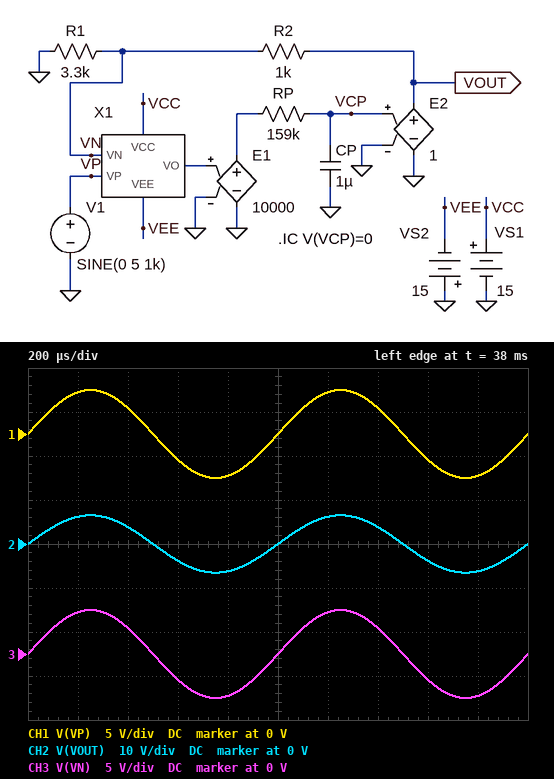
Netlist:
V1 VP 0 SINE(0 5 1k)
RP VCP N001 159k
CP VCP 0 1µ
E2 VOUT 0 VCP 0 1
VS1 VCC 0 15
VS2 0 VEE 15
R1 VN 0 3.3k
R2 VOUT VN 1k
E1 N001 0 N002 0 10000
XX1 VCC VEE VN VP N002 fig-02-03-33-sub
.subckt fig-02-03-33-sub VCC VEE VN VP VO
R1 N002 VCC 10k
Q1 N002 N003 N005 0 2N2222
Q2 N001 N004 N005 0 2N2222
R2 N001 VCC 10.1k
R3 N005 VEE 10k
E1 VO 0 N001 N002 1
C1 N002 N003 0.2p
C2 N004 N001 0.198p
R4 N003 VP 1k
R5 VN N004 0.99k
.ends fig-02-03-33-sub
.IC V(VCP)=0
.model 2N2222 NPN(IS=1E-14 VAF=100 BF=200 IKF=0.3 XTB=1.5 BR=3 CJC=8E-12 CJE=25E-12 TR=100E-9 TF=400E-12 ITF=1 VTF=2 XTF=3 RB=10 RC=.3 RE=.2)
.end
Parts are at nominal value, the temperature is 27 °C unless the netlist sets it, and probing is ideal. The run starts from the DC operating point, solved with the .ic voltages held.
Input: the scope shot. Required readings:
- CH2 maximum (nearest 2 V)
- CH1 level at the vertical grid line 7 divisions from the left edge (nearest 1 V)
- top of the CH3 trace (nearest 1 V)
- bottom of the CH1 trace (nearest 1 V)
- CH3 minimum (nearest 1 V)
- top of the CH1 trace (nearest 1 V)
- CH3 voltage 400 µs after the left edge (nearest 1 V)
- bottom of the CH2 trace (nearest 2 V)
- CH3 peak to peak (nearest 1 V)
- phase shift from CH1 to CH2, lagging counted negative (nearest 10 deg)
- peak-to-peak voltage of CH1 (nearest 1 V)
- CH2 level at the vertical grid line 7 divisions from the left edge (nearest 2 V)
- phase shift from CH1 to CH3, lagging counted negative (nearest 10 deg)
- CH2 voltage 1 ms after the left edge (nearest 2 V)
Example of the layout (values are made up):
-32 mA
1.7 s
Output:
6 V
3 V
5 V
-5 V
-5 V
5 V
3 V
-6 V
10 V
0 deg
10 V
4 V
0 deg
0 V
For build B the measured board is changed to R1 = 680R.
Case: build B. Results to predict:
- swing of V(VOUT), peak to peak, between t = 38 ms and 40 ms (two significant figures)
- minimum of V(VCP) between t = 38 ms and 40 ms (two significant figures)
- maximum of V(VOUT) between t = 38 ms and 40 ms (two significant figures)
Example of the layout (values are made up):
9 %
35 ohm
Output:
25 V
-12 V
12 V
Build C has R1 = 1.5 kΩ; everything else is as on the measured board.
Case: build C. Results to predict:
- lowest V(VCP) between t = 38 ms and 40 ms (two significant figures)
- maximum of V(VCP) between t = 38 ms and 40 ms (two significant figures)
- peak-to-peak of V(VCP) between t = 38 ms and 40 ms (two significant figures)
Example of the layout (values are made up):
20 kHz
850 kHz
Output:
-8.3 V
8.3 V
17 V
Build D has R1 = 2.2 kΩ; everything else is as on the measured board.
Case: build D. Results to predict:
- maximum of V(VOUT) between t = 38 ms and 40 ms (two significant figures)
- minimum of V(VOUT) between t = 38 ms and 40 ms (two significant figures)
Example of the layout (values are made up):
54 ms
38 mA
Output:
7.3 V
-7.3 V
